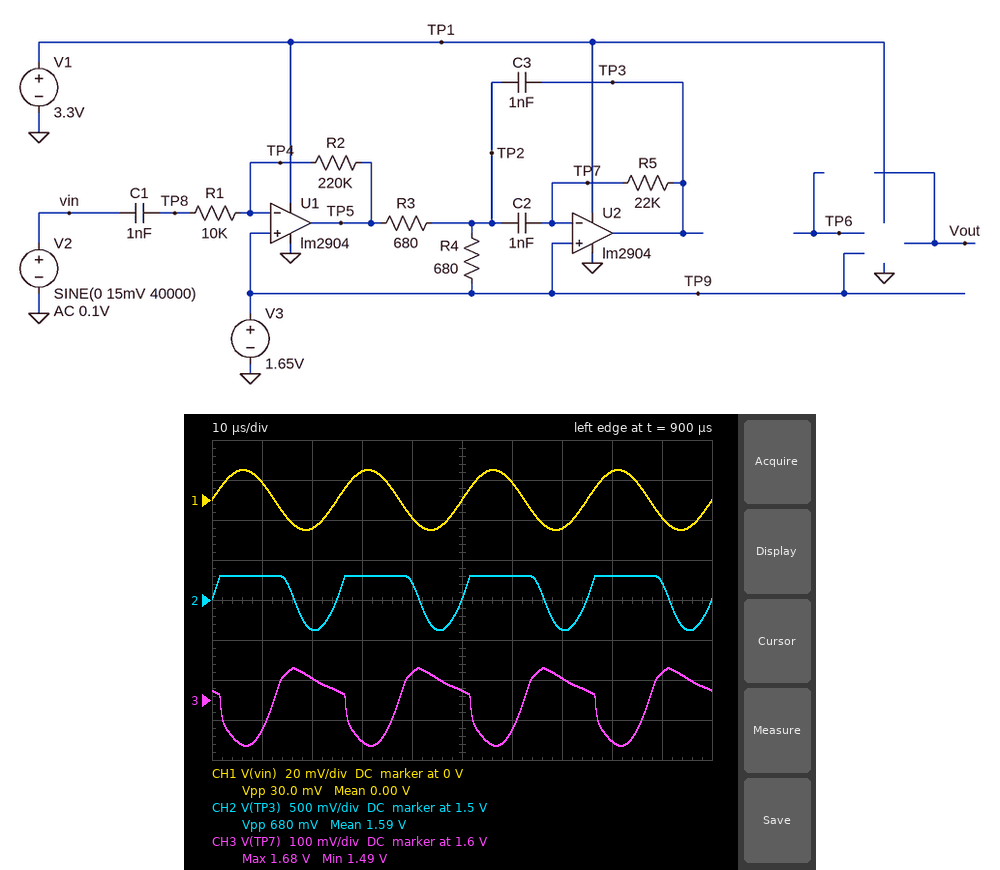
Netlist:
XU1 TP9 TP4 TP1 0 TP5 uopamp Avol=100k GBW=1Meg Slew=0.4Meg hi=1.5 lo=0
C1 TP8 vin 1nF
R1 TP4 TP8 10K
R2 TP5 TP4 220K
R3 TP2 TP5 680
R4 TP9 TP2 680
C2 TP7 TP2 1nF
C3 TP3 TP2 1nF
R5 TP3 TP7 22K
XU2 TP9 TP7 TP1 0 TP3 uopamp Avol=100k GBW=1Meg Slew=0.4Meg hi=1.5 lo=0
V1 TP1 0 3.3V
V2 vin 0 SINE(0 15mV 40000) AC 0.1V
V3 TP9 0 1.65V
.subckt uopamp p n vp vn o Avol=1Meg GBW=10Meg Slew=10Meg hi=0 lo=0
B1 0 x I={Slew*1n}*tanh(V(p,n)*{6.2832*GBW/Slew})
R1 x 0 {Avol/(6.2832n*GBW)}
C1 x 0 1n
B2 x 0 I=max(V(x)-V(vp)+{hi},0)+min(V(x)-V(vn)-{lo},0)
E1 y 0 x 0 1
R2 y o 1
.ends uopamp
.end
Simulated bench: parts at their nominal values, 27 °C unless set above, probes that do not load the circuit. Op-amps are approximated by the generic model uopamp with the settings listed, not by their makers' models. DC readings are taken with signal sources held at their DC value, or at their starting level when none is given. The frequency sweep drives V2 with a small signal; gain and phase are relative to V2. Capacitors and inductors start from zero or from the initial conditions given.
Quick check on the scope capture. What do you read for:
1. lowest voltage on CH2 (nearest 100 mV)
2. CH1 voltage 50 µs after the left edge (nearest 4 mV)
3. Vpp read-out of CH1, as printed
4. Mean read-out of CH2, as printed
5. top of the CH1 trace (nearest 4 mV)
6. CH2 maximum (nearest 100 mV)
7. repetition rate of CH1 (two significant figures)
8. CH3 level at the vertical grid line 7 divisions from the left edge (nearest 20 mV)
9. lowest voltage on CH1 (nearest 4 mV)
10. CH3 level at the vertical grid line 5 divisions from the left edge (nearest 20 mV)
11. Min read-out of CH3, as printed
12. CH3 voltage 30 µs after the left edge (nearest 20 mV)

1.1 V
0 V
30.0 mV
1.59 V
16 mV
1.8 V
40 kHz
1.66 V
-16 mV
1.62 V
1.49 V
1.50 V
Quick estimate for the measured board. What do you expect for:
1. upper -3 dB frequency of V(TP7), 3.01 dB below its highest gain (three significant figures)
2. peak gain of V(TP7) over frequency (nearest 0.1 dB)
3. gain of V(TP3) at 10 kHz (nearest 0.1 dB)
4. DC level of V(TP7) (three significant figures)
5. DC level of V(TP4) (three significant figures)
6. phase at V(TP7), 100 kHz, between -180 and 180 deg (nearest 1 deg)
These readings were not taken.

53.9 kHz
21.9 dB
19.4 dB
1.65 V
1.65 V
119 deg
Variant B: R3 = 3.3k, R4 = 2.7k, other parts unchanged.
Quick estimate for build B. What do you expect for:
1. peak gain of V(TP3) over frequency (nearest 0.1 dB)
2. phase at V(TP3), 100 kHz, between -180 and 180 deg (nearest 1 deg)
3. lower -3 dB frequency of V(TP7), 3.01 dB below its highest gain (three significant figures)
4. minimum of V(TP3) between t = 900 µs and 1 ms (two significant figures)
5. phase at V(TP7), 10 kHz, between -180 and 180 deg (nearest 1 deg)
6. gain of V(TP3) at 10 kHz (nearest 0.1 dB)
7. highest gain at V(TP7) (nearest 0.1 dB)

37.1 dB
-152 deg
22.8 kHz
1.4 V
40 deg
19.3 dB
5.8 dB
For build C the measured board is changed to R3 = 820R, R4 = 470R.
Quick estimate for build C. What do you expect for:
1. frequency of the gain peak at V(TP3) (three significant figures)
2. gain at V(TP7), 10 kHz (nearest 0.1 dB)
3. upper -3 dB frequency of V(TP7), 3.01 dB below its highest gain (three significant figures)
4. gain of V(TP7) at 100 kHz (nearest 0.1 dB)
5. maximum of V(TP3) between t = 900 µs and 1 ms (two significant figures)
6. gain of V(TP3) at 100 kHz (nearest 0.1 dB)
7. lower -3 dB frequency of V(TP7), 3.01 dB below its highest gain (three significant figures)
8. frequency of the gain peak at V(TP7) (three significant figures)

49.7 kHz
-23.4 dB
55.8 kHz
3.8 dB
1.8 V
23.8 dB
45.5 kHz
50.2 kHz
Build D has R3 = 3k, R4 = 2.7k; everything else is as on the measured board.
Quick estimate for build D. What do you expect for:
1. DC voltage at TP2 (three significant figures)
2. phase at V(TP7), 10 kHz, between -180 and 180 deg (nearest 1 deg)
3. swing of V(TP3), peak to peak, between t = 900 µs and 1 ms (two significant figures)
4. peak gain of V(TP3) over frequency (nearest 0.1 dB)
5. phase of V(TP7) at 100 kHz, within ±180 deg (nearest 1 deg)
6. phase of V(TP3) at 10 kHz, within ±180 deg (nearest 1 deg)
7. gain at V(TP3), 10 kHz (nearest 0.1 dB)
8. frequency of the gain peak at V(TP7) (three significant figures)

1.65 V
41 deg
400 mV
37.9 dB
118 deg
131 deg
19.7 dB
28.5 kHz
